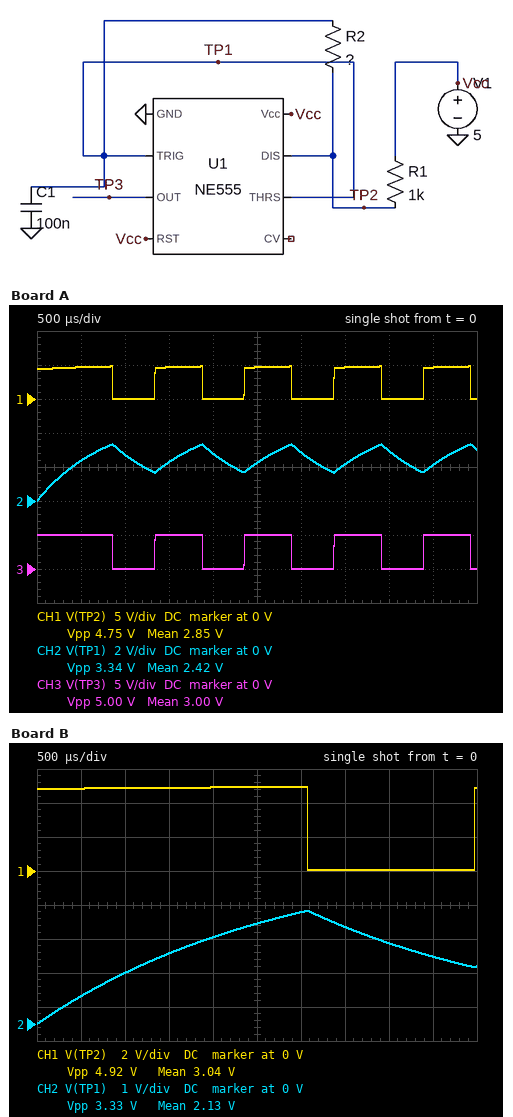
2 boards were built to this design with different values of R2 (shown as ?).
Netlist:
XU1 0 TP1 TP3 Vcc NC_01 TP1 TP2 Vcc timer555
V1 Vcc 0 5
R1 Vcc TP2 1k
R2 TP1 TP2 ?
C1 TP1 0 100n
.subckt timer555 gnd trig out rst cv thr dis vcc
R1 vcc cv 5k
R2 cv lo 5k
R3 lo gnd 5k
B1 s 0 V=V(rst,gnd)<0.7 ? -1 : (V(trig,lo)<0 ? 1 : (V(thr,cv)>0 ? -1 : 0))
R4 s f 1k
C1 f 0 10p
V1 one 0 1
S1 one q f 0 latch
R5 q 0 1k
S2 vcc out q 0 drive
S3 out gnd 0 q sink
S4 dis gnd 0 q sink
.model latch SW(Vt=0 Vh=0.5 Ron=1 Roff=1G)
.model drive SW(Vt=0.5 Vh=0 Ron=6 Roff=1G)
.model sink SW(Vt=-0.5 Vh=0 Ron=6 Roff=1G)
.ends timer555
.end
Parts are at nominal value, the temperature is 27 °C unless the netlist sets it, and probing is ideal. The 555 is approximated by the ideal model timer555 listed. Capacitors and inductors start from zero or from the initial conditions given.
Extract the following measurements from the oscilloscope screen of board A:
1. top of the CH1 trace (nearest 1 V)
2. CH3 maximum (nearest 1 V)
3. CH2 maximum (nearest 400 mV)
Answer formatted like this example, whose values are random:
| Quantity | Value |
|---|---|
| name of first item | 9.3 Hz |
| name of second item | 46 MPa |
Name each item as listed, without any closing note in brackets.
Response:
| Quantity | Value |
|---|---|
| top of the CH1 trace | 5 V |
| CH3 maximum | 5 V |
| CH2 maximum | 3.2 V |
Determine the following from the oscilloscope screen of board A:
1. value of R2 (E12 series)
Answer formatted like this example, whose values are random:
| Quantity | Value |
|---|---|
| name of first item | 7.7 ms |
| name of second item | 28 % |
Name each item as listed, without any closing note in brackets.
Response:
| Quantity | Value |
|---|---|
| value of R2 | 6.8 kΩ |
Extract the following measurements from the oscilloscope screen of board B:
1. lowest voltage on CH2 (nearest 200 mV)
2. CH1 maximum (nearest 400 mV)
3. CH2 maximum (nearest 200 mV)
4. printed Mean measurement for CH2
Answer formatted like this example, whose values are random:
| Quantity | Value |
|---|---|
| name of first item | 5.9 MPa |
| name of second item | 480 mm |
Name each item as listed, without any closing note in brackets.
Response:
| Quantity | Value |
|---|---|
| lowest voltage on CH2 | 0 V |
| CH1 maximum | 4.8 V |
| CH2 maximum | 3.4 V |
| printed Mean measurement for CH2 | 2.13 V |
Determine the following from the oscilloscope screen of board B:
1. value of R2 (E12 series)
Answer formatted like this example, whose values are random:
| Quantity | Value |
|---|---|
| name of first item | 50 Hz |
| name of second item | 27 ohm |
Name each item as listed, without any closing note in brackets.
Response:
| Quantity | Value |
|---|---|
| value of R2 | 27 kΩ |
